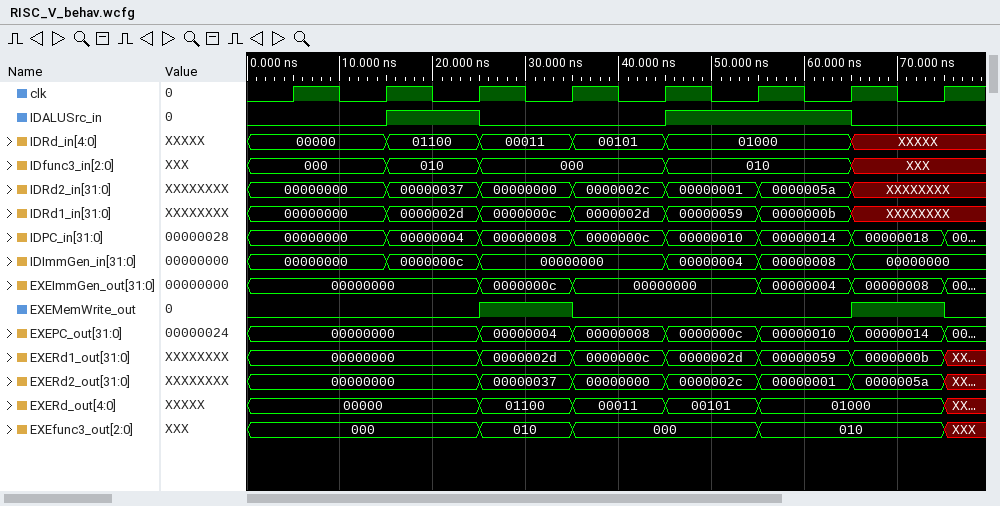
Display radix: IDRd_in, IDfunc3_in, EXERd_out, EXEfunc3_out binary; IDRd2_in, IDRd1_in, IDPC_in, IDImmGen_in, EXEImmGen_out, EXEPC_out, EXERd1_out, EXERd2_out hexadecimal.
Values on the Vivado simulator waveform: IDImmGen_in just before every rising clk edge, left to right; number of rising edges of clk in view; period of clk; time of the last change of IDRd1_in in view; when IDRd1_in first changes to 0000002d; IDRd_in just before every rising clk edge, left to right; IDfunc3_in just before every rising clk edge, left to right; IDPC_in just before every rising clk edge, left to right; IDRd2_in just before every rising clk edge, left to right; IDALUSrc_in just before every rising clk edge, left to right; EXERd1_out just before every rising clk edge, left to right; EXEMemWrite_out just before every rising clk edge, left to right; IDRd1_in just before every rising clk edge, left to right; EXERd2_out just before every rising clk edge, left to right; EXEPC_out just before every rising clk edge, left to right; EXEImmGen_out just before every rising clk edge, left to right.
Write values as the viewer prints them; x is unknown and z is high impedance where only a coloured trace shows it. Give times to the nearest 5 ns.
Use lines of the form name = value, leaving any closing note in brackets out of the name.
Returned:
IDImmGen_in just before every rising clk edge, left to right = 00000000, 00000000, 0000000c, 00000000, 00000000, 00000004, 00000008, 00000000
number of rising edges of clk in view = 8
period of clk = 10 ns
time of the last change of IDRd1_in in view = 65 ns
when IDRd1_in first changes to 0000002d = 15 ns
IDRd_in just before every rising clk edge, left to right = 00000, 00000, 01100, 00011, 00101, 01000, 01000, XXXXX
IDfunc3_in just before every rising clk edge, left to right = 000, 000, 010, 000, 000, 010, 010, XXX
IDPC_in just before every rising clk edge, left to right = 00000000, 00000000, 00000004, 00000008, 0000000c, 00000010, 00000014, 00000018
IDRd2_in just before every rising clk edge, left to right = 00000000, 00000000, 00000037, 00000000, 0000002c, 00000001, 0000005a, XXXXXXXX
IDALUSrc_in just before every rising clk edge, left to right = 0 0 1 0 0 1 1 0
EXERd1_out just before every rising clk edge, left to right = 00000000, 00000000, 00000000, 0000002d, 0000000c, 0000002d, 00000059, 0000000b
EXEMemWrite_out just before every rising clk edge, left to right = 0 0 0 1 0 0 0 1
IDRd1_in just before every rising clk edge, left to right = 00000000, 00000000, 0000002d, 0000000c, 0000002d, 00000059, 0000000b, XXXXXXXX
EXERd2_out just before every rising clk edge, left to right = 00000000, 00000000, 00000000, 00000037, 00000000, 0000002c, 00000001, 0000005a
EXEPC_out just before every rising clk edge, left to right = 00000000, 00000000, 00000000, 00000004, 00000008, 0000000c, 00000010, 00000014
EXEImmGen_out just before every rising clk edge, left to right = 00000000, 00000000, 00000000, 0000000c, 00000000, 00000000, 00000004, 00000008
